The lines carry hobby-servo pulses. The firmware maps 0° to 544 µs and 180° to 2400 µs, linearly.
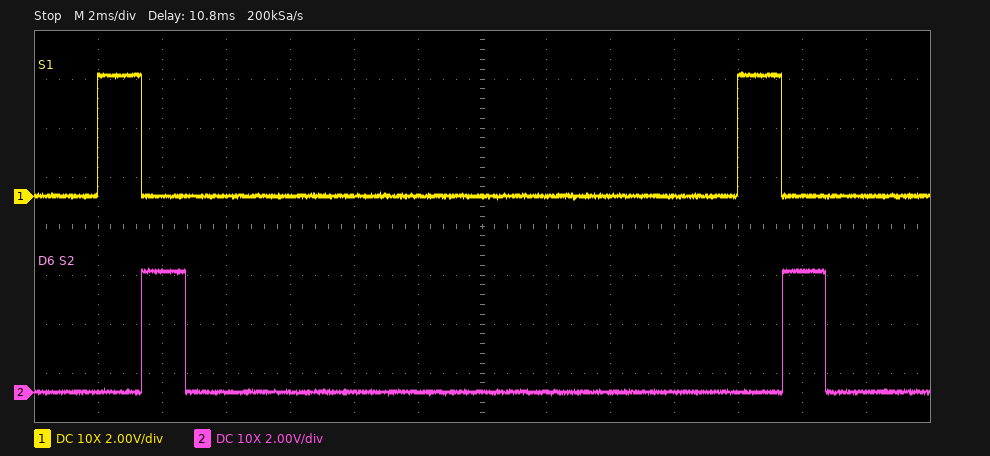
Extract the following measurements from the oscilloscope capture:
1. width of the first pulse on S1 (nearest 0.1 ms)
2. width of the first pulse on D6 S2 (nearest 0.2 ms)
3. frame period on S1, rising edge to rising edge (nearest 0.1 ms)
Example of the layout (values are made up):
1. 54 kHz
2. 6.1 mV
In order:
1. 1.4 ms
2. 1.4 ms
3. 20.0 ms
